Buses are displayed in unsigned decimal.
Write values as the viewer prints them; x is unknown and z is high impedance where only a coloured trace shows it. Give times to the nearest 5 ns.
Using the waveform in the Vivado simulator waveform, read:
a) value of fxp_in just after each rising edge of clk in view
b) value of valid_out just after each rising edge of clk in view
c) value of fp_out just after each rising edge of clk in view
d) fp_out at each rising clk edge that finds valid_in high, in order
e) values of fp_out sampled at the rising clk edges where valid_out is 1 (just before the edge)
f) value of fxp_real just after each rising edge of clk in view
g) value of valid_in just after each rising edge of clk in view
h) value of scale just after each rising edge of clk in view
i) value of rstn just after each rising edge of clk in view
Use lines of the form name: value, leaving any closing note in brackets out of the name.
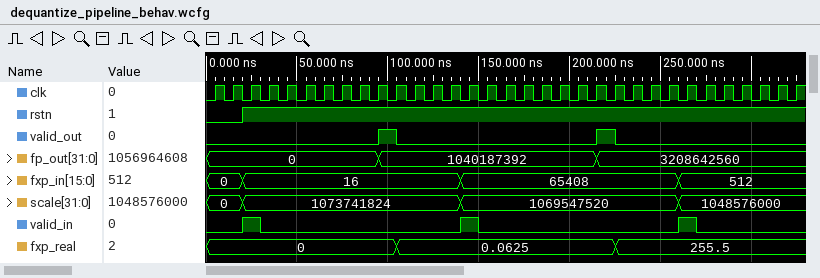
value of fxp_in just after each rising edge of clk in view: 0, 0, 16, 16, 16, 16, 16, 16, 16, 16, 16, 16, 16, 16, 65408, 65408, 65408, 65408, 65408, 65408, 65408, 65408, 65408, 65408, 65408, 65408, 512, 512, 512, 512, 512, 512, 512
value of valid_out just after each rising edge of clk in view: 0 0 0 0 0 0 0 0 0 1 0 0 0 0 0 0 0 0 0 0 0 1 0 0 0 0 0 0 0 0 0 0 0
value of fp_out just after each rising edge of clk in view: 0, 0, 0, 0, 0, 0, 0, 0, 0, 1040187392, 1040187392, 1040187392, 1040187392, 1040187392, 1040187392, 1040187392, 1040187392, 1040187392, 1040187392, 1040187392, 1040187392, 3208642560, 3208642560, 3208642560, 3208642560, 3208642560, 3208642560, 3208642560, 3208642560, 3208642560, 3208642560, 3208642560, 3208642560
fp_out at each rising clk edge that finds valid_in high, in order: 0, 1040187392, 3208642560
values of fp_out sampled at the rising clk edges where valid_out is 1: 1040187392, 3208642560
value of fxp_real just after each rising edge of clk in view: 0, 0, 0, 0, 0, 0, 0, 0, 0, 0, 0.0625, 0.0625, 0.0625, 0.0625, 0.0625, 0.0625, 0.0625, 0.0625, 0.0625, 0.0625, 0.0625, 0.0625, 255.5, 255.5, 255.5, 255.5, 255.5, 255.5, 255.5, 255.5, 255.5, 255.5, 255.5
value of valid_in just after each rising edge of clk in view: 0 0 1 0 0 0 0 0 0 0 0 0 0 0 1 0 0 0 0 0 0 0 0 0 0 0 1 0 0 0 0 0 0
value of scale just after each rising edge of clk in view: 0, 0, 1073741824, 1073741824, 1073741824, 1073741824, 1073741824, 1073741824, 1073741824, 1073741824, 1073741824, 1073741824, 1073741824, 1073741824, 1069547520, 1069547520, 1069547520, 1069547520, 1069547520, 1069547520, 1069547520, 1069547520, 1069547520, 1069547520, 1069547520, 1069547520, 1048576000, 1048576000, 1048576000, 1048576000, 1048576000, 1048576000, 1048576000
value of rstn just after each rising edge of clk in view: 0 0 1 1 1 1 1 1 1 1 1 1 1 1 1 1 1 1 1 1 1 1 1 1 1 1 1 1 1 1 1 1 1
